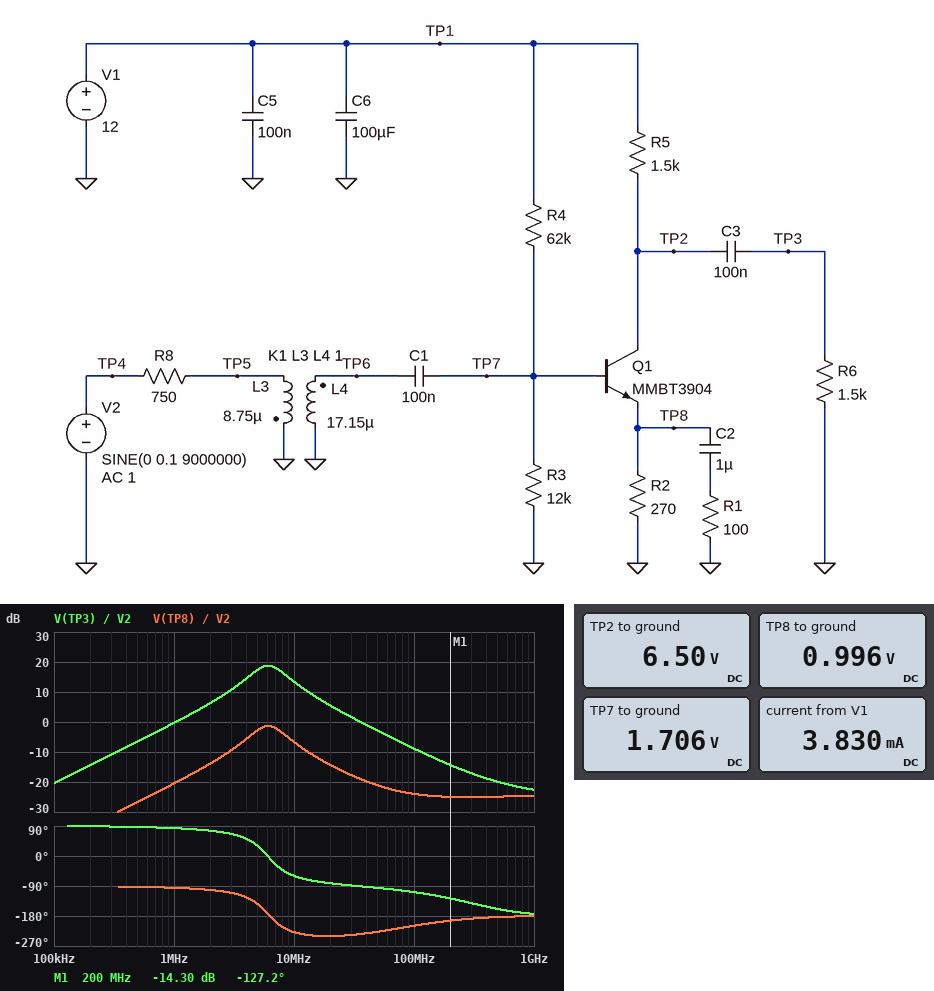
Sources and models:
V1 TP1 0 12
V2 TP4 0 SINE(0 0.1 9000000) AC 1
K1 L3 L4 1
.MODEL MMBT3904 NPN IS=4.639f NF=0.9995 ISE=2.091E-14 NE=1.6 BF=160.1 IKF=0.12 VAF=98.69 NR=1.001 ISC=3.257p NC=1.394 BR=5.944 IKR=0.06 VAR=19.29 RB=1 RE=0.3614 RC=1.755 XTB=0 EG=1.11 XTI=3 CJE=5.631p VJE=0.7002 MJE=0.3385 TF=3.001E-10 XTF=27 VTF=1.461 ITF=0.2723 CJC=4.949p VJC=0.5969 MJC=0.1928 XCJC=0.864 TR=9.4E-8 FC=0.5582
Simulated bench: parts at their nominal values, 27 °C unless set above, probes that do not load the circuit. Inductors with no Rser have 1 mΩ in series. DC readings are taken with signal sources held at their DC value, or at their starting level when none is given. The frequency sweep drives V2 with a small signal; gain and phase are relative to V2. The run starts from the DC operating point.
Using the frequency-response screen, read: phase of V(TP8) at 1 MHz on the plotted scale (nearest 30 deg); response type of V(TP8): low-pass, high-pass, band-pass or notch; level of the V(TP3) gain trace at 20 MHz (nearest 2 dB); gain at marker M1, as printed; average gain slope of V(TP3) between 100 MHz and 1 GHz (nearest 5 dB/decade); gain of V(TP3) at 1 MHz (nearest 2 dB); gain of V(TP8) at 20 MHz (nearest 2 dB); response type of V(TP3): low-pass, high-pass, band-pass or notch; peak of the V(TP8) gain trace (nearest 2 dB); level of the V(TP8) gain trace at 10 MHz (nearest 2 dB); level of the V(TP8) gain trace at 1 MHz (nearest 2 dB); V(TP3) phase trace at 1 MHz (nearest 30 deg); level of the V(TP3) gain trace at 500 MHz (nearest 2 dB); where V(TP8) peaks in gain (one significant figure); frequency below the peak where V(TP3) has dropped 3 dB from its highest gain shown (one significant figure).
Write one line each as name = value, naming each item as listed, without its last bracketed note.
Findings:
phase of V(TP8) at 1 MHz on the plotted scale = -90 deg
response type of V(TP8): low-pass, high-pass, band-pass or notch = band-pass
level of the V(TP3) gain trace at 20 MHz = 6 dB
gain at marker M1, as printed = -14.30 dB
average gain slope of V(TP3) between 100 MHz and 1 GHz = -15 dB/decade
gain of V(TP3) at 1 MHz = 0 dB
gain of V(TP8) at 20 MHz = -14 dB
response type of V(TP3): low-pass, high-pass, band-pass or notch = band-pass
peak of the V(TP8) gain trace = -2 dB
level of the V(TP8) gain trace at 10 MHz = -6 dB
level of the V(TP8) gain trace at 1 MHz = -20 dB
V(TP3) phase trace at 1 MHz = 90 deg
level of the V(TP3) gain trace at 500 MHz = -20 dB
where V(TP8) peaks in gain = 6 MHz
frequency below the peak where V(TP3) has dropped 3 dB from its highest gain shown = 4 MHz
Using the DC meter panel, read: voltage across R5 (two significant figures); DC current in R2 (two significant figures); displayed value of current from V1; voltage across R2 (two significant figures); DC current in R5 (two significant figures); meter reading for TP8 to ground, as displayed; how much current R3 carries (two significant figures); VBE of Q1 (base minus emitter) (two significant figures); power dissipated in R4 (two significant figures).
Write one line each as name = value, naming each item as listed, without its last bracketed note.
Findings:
voltage across R5 = 5.5 V
DC current in R2 = 3.7 mA
displayed value of current from V1 = 3.830 mA
voltage across R2 = 1.0 V
DC current in R5 = 3.7 mA
meter reading for TP8 to ground, as displayed = 0.996 V
how much current R3 carries = 140 µA
VBE of Q1 (base minus emitter) = 710 mV
power dissipated in R4 = 1.7 mW
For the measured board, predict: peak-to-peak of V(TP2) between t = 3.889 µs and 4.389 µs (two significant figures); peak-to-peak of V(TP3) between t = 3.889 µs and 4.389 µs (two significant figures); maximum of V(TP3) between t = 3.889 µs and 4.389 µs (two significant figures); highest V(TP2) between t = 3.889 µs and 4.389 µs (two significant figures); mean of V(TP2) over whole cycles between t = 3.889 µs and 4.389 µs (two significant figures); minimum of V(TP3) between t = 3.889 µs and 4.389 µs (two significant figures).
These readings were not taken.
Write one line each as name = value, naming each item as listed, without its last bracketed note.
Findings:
peak-to-peak of V(TP2) between t = 3.889 µs and 4.389 µs = 1.1 V
peak-to-peak of V(TP3) between t = 3.889 µs and 4.389 µs = 1.1 V
maximum of V(TP3) between t = 3.889 µs and 4.389 µs = 550 mV
highest V(TP2) between t = 3.889 µs and 4.389 µs = 7.1 V
mean of V(TP2) over whole cycles between t = 3.889 µs and 4.389 µs = 6.5 V
minimum of V(TP3) between t = 3.889 µs and 4.389 µs = -550 mV
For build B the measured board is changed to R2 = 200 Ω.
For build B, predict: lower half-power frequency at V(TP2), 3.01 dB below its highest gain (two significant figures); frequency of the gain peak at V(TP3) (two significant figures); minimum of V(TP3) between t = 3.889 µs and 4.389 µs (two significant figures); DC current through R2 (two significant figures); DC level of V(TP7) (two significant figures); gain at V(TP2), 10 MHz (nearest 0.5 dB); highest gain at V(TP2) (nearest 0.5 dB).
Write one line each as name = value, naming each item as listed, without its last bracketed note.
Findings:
lower half-power frequency at V(TP2), 3.01 dB below its highest gain = 4.2 MHz
frequency of the gain peak at V(TP3) = 5.7 MHz
minimum of V(TP3) between t = 3.889 µs and 4.389 µs = -520 mV
DC current through R2 = 4.6 mA
DC level of V(TP7) = 1.6 V
gain at V(TP2), 10 MHz = 13.0 dB
highest gain at V(TP2) = 19.5 dB
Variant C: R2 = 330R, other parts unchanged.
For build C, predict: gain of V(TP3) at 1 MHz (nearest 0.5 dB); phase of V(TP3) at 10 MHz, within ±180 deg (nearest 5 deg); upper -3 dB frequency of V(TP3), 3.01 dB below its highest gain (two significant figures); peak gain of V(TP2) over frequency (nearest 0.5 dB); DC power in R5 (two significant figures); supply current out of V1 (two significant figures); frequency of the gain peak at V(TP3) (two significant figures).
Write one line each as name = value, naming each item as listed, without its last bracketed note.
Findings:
gain of V(TP3) at 1 MHz = -1.0 dB
phase of V(TP3) at 10 MHz, within ±180 deg = -55 deg
upper -3 dB frequency of V(TP3), 3.01 dB below its highest gain = 8.8 MHz
peak gain of V(TP2) over frequency = 18.5 dB
DC power in R5 = 15 mW
supply current out of V1 = 3.3 mA
frequency of the gain peak at V(TP3) = 6.3 MHz
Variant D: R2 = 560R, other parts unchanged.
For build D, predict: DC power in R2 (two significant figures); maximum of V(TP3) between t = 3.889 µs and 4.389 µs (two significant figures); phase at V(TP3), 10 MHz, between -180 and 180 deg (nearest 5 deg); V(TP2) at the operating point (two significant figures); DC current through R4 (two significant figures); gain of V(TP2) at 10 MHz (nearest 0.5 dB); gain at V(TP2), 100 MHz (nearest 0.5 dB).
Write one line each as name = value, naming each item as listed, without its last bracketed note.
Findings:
DC power in R2 = 2.3 mW
maximum of V(TP3) between t = 3.889 µs and 4.389 µs = 560 mV
phase at V(TP3), 10 MHz, between -180 and 180 deg = -50 deg
V(TP2) at the operating point = 9.0 V
DC current through R4 = 160 µA
gain of V(TP2) at 10 MHz = 14.0 dB
gain at V(TP2), 100 MHz = -8.5 dB
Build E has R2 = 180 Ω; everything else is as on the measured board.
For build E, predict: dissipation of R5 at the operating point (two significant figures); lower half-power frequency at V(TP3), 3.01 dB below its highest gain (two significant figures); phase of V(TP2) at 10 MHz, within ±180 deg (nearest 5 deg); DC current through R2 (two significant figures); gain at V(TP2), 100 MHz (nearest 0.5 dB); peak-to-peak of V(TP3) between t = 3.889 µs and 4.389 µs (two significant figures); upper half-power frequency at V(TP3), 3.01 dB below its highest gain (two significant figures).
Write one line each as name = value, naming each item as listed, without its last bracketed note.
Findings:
dissipation of R5 at the operating point = 37 mW
lower half-power frequency at V(TP3), 3.01 dB below its highest gain = 4.1 MHz
phase of V(TP2) at 10 MHz, within ±180 deg = -65 deg
DC current through R2 = 5.0 mA
gain at V(TP2), 100 MHz = -9.5 dB
peak-to-peak of V(TP3) between t = 3.889 µs and 4.389 µs = 1.0 V
upper half-power frequency at V(TP3), 3.01 dB below its highest gain = 7.5 MHz
